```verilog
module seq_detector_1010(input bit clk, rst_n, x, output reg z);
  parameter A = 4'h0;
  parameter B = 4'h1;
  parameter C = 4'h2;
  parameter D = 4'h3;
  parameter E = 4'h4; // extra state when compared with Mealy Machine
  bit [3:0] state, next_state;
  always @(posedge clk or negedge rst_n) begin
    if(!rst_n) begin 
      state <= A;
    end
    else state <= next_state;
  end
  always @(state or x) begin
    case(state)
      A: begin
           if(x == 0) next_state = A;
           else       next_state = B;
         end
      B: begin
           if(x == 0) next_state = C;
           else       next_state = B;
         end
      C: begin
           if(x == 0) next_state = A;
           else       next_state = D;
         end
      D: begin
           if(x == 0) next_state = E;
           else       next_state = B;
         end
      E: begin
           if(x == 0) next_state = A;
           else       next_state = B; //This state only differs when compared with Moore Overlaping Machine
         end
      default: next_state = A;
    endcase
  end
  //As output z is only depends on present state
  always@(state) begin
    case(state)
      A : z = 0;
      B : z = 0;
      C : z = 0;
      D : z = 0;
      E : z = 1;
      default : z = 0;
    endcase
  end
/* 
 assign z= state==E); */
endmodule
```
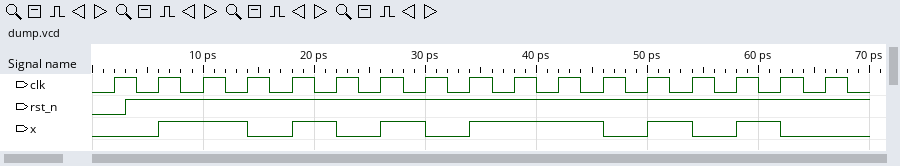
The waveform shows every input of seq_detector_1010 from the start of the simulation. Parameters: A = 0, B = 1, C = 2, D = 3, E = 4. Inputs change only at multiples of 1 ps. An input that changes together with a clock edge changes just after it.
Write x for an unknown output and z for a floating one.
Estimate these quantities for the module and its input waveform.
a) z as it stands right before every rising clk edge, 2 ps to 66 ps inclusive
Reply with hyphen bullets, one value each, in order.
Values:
- x x x 0 0 0 0 1 0 0 0 0 0 0 0 1 0
